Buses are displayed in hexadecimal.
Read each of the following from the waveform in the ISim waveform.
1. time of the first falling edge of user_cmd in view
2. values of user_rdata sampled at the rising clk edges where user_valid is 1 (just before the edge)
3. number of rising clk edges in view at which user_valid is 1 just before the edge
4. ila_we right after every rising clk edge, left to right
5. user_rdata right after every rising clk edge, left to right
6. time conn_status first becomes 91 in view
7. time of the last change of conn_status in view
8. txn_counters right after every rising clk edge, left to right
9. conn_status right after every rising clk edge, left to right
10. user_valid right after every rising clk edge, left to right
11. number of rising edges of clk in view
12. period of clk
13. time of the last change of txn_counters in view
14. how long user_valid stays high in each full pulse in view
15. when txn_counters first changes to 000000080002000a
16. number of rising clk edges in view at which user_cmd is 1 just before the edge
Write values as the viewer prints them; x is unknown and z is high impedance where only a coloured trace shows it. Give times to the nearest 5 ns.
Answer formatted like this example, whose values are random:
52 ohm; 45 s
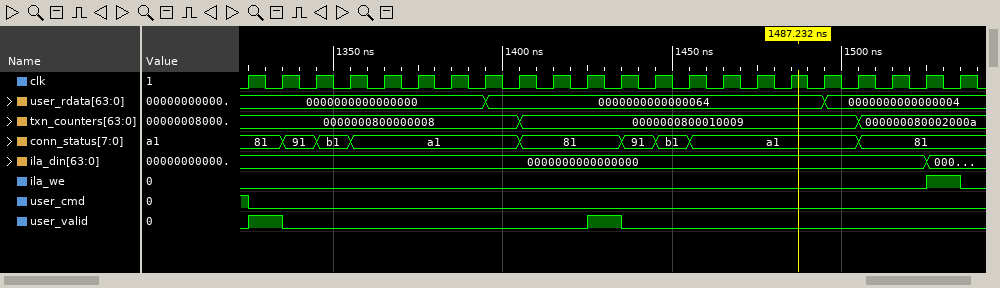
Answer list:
1325 ns; 0000000000000000, 0000000000000064; 2; 0 0 0 0 0 0 0 0 0 0 0 0 0 0 0 0 0 0 0 0 1 0; 0000000000000000, 0000000000000000, 0000000000000000, 0000000000000000, 0000000000000000, 0000000000000000, 0000000000000000, 0000000000000064, 0000000000000064, 0000000000000064, 0000000000000064, 0000000000000064, 0000000000000064, 0000000000000064, 0000000000000064, 0000000000000064, 0000000000000064, 0000000000000004, 0000000000000004, 0000000000000004, 0000000000000004, 0000000000000004; 1335 ns; 1505 ns; 0000000800000008, 0000000800000008, 0000000800000008, 0000000800000008, 0000000800000008, 0000000800000008, 0000000800000008, 0000000800000008, 0000000800010009, 0000000800010009, 0000000800010009, 0000000800010009, 0000000800010009, 0000000800010009, 0000000800010009, 0000000800010009, 0000000800010009, 0000000800010009, 000000080002000a, 000000080002000a, 000000080002000a, 000000080002000a; 81, 91, b1, a1, a1, a1, a1, a1, 81, 81, 81, 91, b1, a1, a1, a1, a1, a1, 81, 81, 81, 81; 1 0 0 0 0 0 0 0 0 0 1 0 0 0 0 0 0 0 0 0 0 0; 22; 10 ns; 1505 ns; 10 ns, 10 ns; 1505 ns; 1
